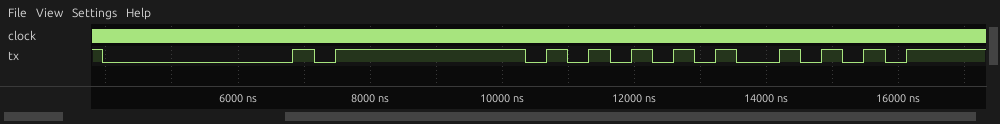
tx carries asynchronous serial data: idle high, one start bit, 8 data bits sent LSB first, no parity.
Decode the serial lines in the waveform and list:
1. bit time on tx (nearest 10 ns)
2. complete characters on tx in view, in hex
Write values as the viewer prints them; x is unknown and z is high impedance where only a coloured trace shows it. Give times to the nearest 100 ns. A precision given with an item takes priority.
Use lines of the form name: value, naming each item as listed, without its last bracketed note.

bit time on tx: 320 ns
complete characters on tx in view, in hex: 00, FF, 55, AA
